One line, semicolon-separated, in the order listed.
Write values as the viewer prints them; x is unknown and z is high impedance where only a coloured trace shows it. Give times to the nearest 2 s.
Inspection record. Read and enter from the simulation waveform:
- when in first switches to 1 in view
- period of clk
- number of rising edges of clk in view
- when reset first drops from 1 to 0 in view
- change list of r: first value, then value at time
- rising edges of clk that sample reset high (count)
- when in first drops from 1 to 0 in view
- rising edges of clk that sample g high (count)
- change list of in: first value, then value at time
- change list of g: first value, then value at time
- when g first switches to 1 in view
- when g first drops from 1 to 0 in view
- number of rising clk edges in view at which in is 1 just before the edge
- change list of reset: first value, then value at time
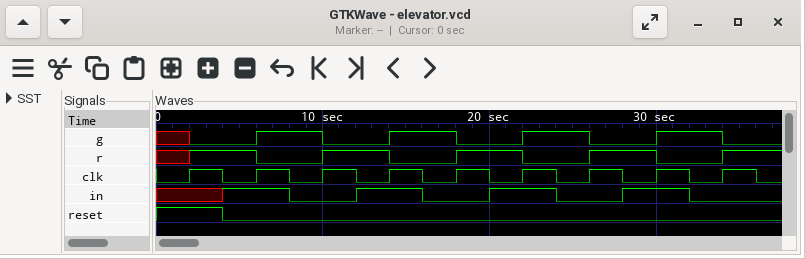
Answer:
4 s; 4 s; 9; 4 s; x, 1 at 2 s, 0 at 6 s, 1 at 10 s, 0 at 14 s, 1 at 18 s, 0 at 22 s, 1 at 26 s, 0 at 30 s, 1 at 34 s; 1; 8 s; 4; x, 1 at 4 s, 0 at 8 s, 1 at 12 s, 0 at 16 s, 1 at 20 s, 0 at 24 s, 1 at 28 s, 0 at 32 s; x, 0 at 2 s, 1 at 6 s, 0 at 10 s, 1 at 14 s, 0 at 18 s, 1 at 22 s, 0 at 26 s, 1 at 30 s, 0 at 34 s; 6 s; 10 s; 4; 1, 0 at 4 s
